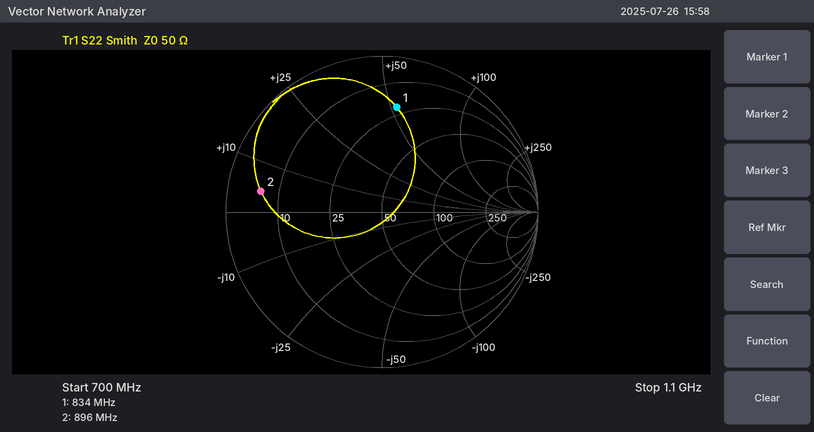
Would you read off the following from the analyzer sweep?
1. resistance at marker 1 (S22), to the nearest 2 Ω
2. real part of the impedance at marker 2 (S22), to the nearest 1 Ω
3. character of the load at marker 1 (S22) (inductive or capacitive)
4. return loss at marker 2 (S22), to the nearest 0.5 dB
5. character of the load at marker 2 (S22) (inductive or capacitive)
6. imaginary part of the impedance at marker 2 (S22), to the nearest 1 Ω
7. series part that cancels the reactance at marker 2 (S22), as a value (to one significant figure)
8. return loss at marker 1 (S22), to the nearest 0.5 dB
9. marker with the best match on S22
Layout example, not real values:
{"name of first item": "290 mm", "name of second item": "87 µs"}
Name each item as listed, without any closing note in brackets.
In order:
{"resistance at marker 1 (S22), to the nearest 2 Ω": "22 Ω", "real part of the impedance at marker 2 (S22), to the nearest 1 Ω": "6 Ω", "character of the load at marker 1 (S22)": "inductive", "return loss at marker 2 (S22), to the nearest 0.5 dB": "2.0 dB", "character of the load at marker 2 (S22)": "inductive", "imaginary part of the impedance at marker 2 (S22), to the nearest 1 Ω": "+4 Ω", "series part that cancels the reactance at marker 2 (S22), as a value": "40 pF", "return loss at marker 1 (S22), to the nearest 0.5 dB": "3.5 dB", "marker with the best match on S22": "marker 1"}
